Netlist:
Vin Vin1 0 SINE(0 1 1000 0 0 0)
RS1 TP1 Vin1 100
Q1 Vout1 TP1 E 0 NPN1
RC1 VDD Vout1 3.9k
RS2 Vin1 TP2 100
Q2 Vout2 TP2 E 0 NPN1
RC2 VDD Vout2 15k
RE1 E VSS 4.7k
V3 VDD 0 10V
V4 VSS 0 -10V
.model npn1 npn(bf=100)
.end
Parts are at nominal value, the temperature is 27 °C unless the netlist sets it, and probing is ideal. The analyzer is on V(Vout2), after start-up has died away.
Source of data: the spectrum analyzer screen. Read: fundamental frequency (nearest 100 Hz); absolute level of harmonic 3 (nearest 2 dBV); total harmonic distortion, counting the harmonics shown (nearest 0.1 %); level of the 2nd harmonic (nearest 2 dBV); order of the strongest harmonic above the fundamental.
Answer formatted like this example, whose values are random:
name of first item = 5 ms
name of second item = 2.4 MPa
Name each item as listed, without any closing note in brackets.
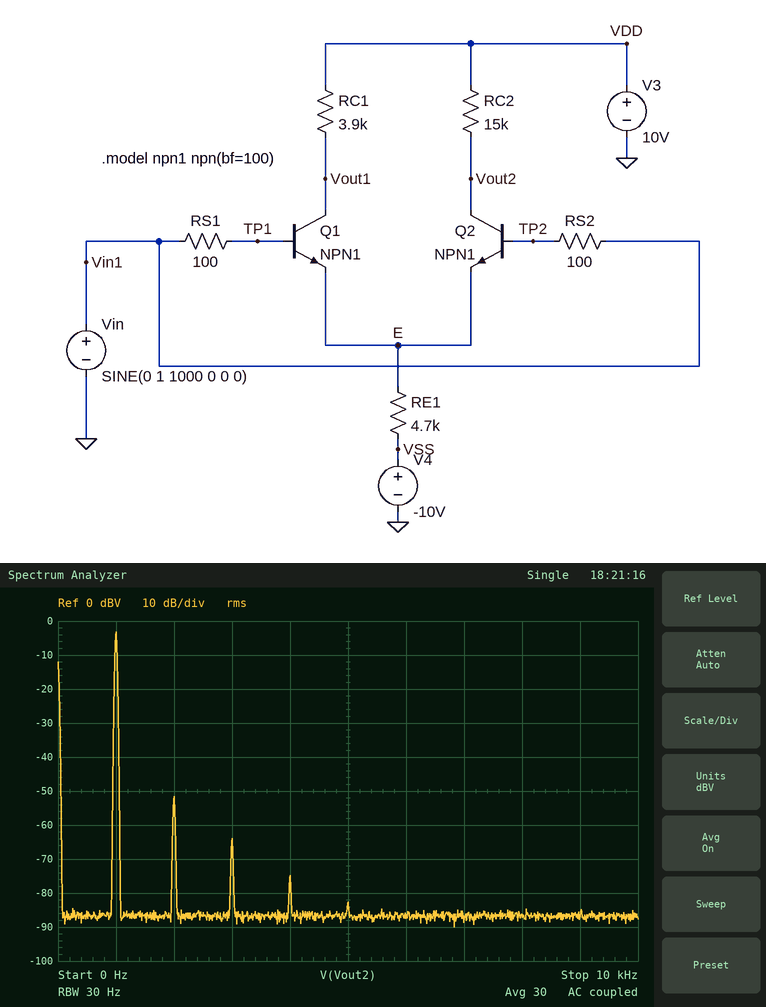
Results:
fundamental frequency = 1.0 kHz
absolute level of harmonic 3 = -64 dBV
total harmonic distortion, counting the harmonics shown = 0.4 %
level of the 2nd harmonic = -52 dBV
order of the strongest harmonic above the fundamental = 2
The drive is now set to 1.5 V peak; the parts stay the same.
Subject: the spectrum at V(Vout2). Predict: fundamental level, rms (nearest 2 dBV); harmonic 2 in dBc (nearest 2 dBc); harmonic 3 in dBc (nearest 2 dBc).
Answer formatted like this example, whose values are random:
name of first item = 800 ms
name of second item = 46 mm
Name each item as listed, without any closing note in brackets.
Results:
fundamental level, rms = 0 dBV
harmonic 2 in dBc = -38 dBc
harmonic 3 in dBc = -44 dBc
